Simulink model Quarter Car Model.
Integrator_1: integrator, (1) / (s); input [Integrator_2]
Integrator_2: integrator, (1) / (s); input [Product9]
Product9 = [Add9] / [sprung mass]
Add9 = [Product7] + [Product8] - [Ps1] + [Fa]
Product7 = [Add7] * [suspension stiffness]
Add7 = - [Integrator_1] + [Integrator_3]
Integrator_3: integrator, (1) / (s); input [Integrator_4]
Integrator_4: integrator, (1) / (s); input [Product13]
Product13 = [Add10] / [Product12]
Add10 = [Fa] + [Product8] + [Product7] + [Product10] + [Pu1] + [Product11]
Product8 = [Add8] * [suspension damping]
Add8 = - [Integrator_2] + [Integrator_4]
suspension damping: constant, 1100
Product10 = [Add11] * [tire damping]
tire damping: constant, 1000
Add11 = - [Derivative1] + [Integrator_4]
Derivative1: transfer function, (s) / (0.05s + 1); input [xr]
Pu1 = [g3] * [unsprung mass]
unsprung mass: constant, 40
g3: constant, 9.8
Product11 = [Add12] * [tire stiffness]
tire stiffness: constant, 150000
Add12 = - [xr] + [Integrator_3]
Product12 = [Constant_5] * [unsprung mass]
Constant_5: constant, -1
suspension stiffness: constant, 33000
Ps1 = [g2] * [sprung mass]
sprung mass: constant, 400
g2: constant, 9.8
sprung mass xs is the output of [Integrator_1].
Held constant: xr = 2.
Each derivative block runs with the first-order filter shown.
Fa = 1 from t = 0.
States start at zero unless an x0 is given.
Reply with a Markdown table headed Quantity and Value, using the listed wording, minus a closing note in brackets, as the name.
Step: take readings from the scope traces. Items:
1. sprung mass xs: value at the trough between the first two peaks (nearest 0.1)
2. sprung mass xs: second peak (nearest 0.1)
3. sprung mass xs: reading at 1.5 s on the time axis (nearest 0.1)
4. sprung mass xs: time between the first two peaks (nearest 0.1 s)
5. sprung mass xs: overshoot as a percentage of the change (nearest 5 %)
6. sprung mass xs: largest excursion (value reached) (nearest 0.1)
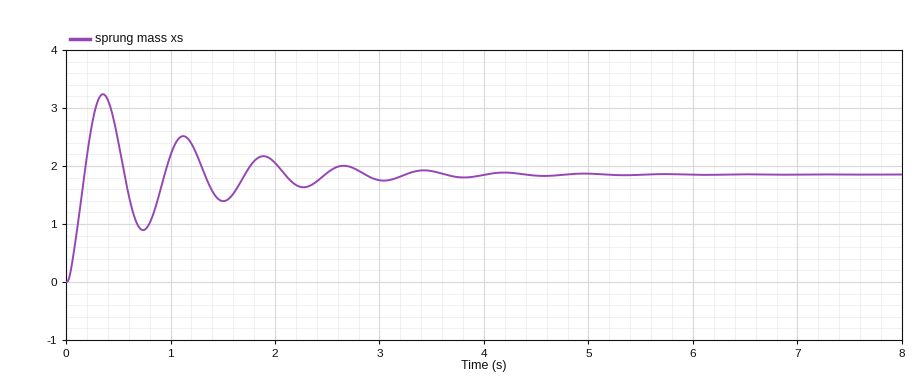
| Quantity | Value |
|---|---|
| sprung mass xs: value at the trough between the first two peaks | 0.9 |
| sprung mass xs: second peak | 2.5 |
| sprung mass xs: reading at 1.5 s on the time axis | 1.4 |
| sprung mass xs: time between the first two peaks | 0.8 s |
| sprung mass xs: overshoot as a percentage of the change | 75 % |
| sprung mass xs: largest excursion (value reached) | 3.2 |
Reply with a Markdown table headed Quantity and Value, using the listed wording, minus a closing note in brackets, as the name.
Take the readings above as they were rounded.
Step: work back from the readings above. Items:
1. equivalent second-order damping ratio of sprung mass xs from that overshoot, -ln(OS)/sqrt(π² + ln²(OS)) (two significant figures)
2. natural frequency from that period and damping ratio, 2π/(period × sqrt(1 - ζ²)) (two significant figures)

| Quantity | Value |
|---|---|
| equivalent second-order damping ratio of sprung mass xs from that overshoot, -ln(OS)/sqrt(π² + ln²(OS)) | 0.091 |
| natural frequency from that period and damping ratio, 2π/(period × sqrt(1 - ζ²)) | 7.9 rad/s |
